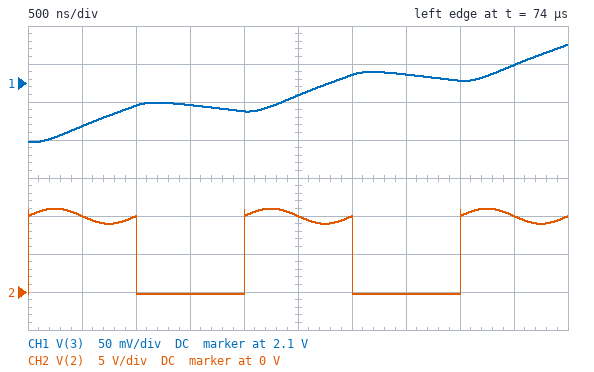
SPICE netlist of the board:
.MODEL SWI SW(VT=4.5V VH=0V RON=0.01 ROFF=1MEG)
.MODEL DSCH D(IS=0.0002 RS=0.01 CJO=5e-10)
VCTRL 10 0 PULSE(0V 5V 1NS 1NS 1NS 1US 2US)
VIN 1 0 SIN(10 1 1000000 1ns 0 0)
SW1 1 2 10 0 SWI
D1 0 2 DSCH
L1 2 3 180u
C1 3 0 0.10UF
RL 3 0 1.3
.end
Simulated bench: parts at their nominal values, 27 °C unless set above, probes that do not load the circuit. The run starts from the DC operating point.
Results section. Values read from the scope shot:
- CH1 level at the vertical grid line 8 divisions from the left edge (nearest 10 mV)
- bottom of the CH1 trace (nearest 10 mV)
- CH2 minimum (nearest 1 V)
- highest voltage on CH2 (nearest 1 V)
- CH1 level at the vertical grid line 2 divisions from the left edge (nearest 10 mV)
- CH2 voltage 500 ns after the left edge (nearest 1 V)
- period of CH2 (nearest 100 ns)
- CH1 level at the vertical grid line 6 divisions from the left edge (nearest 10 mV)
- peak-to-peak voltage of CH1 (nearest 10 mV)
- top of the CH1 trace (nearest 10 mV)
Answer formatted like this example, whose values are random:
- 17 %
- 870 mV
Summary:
- 2.10 V
- 2.02 V
- 0 V
- 11 V
- 2.07 V
- 10 V
- 2.0 µs
- 2.11 V
- 130 mV
- 2.15 V
